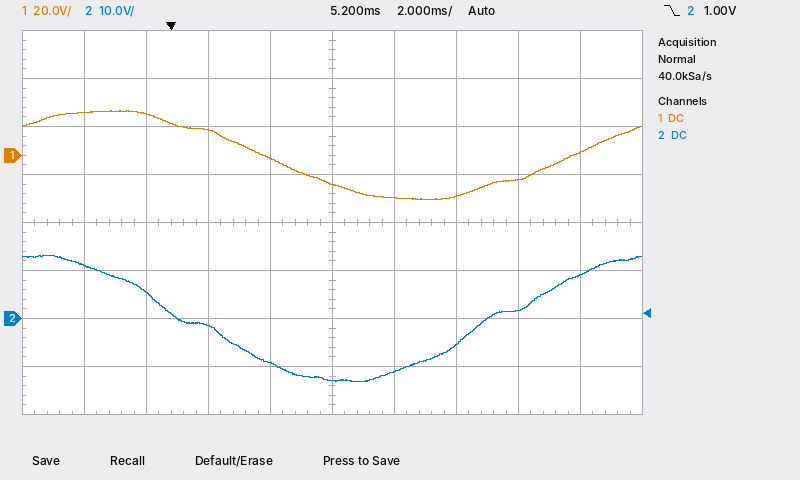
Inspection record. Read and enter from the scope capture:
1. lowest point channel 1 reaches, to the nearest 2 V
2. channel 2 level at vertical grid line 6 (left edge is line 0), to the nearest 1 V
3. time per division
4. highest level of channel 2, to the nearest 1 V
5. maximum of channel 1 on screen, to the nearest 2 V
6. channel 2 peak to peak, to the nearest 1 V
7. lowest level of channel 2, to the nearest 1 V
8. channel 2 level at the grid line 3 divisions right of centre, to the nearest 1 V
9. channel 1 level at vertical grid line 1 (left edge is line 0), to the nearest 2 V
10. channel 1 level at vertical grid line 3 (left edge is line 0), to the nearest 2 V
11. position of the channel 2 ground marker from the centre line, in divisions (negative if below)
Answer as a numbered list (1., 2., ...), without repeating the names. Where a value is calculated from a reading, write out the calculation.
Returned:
1. -18 V
2. -11 V
3. 2 ms
4. 13 V
5. 18 V
6. 13 V − (-13 V) = 26 V
7. -13 V
8. 2 V
9. 18 V
10. 10 V
11. -2.0 div
